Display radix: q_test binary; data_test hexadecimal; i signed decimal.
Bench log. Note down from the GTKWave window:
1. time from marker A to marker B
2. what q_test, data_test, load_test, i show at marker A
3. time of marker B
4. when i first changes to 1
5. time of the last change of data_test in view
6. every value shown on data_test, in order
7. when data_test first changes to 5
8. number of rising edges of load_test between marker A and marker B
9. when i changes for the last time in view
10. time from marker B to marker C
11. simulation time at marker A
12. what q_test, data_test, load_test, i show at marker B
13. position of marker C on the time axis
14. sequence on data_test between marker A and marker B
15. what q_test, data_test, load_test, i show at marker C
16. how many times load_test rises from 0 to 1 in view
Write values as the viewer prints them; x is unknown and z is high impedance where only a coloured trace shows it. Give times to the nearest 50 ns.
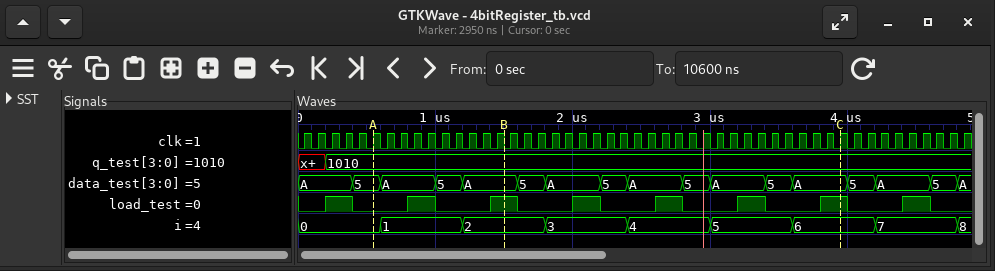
950 ns
q_test=1010, data_test=5, load_test=0, i=0
1500 ns
600 ns
4800 ns
A, 5, A, 5, A, 5, A, 5, A, 5, A, 5, A, 5, A, 5, A
400 ns
2
4800 ns
2450 ns
550 ns
q_test=1010, data_test=A, load_test=1, i=2
3950 ns
5, A, 5, A
q_test=1010, data_test=A, load_test=1, i=6
8
